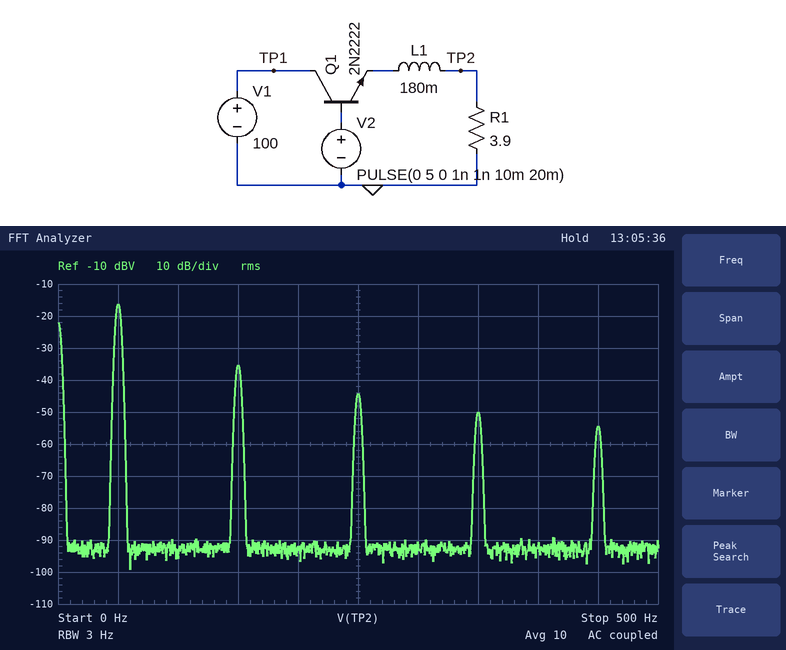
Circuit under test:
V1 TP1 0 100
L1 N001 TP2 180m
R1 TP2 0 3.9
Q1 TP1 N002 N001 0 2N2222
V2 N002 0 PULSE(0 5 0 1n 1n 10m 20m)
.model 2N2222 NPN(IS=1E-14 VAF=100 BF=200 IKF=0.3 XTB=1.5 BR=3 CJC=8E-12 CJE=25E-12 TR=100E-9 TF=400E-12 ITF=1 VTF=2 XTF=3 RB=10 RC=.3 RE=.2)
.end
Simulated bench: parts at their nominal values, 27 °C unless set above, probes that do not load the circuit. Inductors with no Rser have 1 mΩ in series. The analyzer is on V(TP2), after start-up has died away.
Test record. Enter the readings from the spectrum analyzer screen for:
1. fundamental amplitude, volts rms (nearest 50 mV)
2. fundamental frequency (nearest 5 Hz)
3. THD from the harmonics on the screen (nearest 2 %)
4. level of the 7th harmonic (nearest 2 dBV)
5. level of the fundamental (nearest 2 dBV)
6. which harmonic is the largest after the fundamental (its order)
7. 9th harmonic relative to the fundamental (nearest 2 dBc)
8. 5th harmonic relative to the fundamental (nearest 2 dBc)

150 mV
50 Hz
12 %
-50 dBV
-16 dBV
3
-38 dBc
-28 dBc
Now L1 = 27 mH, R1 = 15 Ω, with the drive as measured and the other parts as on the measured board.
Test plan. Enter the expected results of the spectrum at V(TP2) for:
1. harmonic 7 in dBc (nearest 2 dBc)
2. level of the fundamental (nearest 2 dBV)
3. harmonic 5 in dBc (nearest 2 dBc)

-28 dBc
4 dBV
-22 dBc
